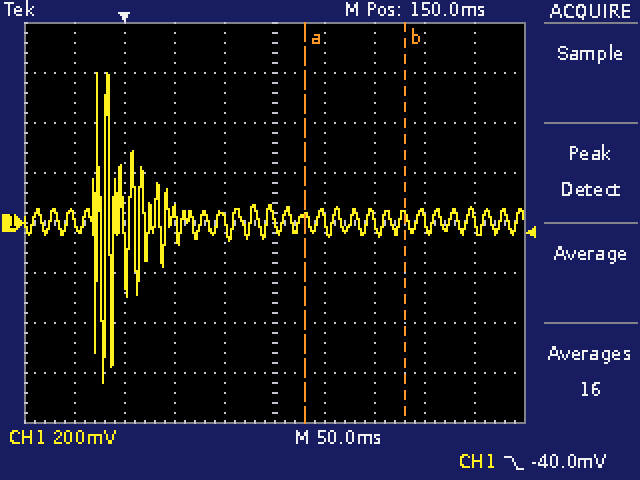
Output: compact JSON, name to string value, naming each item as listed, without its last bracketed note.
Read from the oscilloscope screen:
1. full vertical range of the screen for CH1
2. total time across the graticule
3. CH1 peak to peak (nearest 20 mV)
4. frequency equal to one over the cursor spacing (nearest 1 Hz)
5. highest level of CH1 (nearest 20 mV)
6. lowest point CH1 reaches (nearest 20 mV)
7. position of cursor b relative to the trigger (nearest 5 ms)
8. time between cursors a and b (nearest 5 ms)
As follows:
{"full vertical range of the screen for CH1": "1.6 V", "total time across the graticule": "500 ms", "CH1 peak to peak": "1.24 V", "frequency equal to one over the cursor spacing": "10 Hz", "highest level of CH1": "600 mV", "lowest point CH1 reaches": "-640 mV", "position of cursor b relative to the trigger": "+280 ms", "time between cursors a and b": "100 ms"}
